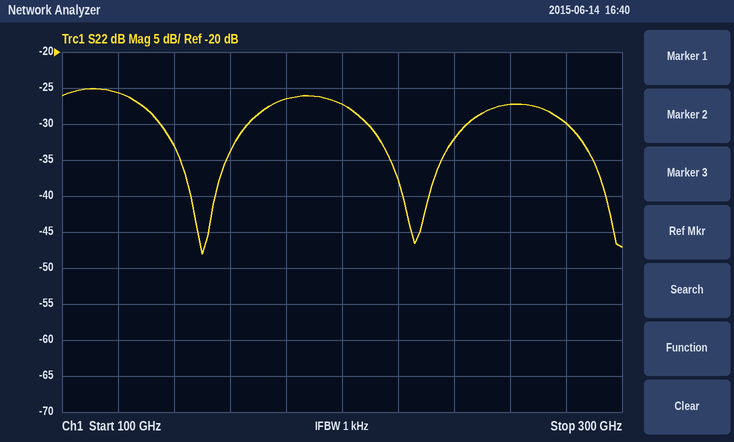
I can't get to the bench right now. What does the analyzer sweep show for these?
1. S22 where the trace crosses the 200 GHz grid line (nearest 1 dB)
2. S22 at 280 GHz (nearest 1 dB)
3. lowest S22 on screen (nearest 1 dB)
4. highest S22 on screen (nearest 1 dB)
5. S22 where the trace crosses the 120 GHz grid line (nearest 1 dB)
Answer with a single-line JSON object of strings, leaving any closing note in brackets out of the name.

{"S22 where the trace crosses the 200 GHz grid line": "-27 dB", "S22 at 280 GHz": "-30 dB", "lowest S22 on screen": "-48 dB", "highest S22 on screen": "-25 dB", "S22 where the trace crosses the 120 GHz grid line": "-26 dB"}
